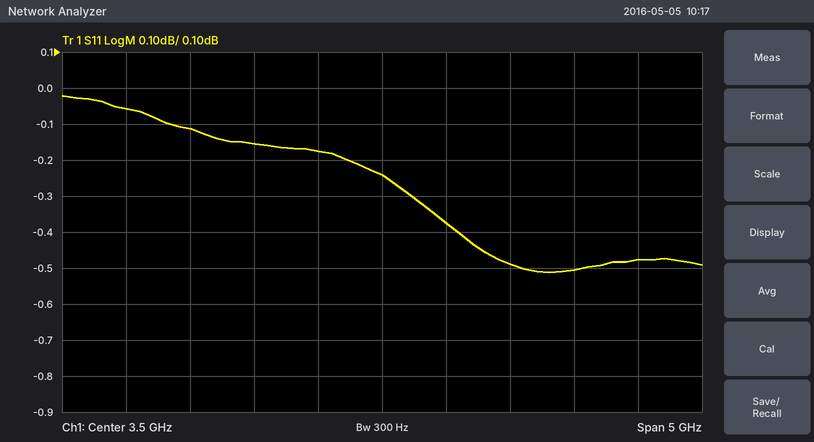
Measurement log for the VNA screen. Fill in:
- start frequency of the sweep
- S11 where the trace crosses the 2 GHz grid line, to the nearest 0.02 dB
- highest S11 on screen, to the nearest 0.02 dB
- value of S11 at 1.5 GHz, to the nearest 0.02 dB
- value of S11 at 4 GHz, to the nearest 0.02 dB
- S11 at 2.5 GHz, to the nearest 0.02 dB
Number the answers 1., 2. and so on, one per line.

1. 1 GHz
2. -0.12 dB
3. -0.02 dB
4. -0.06 dB
5. -0.38 dB
6. -0.16 dB
